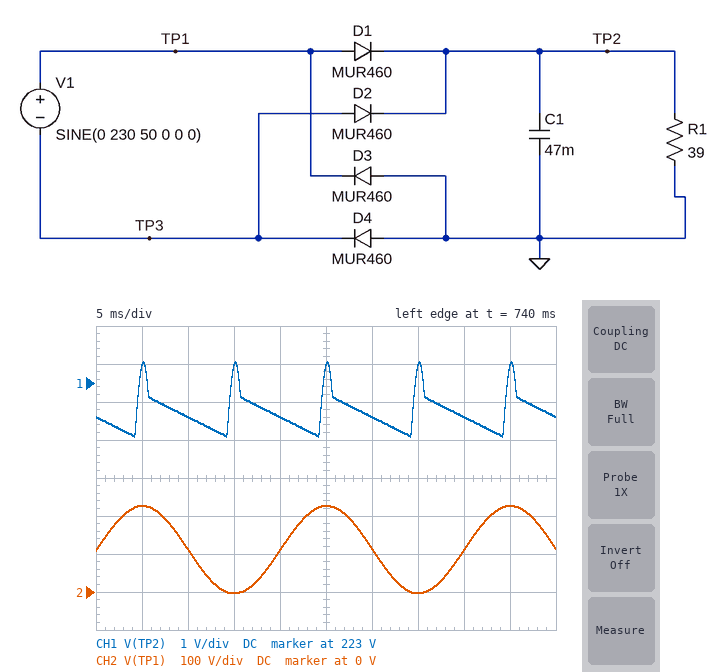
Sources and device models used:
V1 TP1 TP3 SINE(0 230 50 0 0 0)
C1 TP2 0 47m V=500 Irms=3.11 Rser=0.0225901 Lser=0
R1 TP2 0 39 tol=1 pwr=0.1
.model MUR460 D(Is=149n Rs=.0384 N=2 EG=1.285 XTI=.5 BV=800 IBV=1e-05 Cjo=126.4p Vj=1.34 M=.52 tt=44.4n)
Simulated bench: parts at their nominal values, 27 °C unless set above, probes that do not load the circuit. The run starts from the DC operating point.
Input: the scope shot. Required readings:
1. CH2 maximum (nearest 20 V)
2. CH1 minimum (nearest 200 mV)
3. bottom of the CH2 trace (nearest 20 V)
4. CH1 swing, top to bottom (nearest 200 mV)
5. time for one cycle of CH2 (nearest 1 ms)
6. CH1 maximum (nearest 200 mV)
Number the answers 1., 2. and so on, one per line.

1. 220 V
2. 221.6 V
3. 0 V
4. 2.0 V
5. 20 ms
6. 223.6 V
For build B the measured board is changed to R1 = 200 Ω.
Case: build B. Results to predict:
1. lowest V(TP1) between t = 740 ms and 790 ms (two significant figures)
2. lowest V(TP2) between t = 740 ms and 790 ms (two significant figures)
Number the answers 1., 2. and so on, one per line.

1. -1.7 V
2. 230 V
